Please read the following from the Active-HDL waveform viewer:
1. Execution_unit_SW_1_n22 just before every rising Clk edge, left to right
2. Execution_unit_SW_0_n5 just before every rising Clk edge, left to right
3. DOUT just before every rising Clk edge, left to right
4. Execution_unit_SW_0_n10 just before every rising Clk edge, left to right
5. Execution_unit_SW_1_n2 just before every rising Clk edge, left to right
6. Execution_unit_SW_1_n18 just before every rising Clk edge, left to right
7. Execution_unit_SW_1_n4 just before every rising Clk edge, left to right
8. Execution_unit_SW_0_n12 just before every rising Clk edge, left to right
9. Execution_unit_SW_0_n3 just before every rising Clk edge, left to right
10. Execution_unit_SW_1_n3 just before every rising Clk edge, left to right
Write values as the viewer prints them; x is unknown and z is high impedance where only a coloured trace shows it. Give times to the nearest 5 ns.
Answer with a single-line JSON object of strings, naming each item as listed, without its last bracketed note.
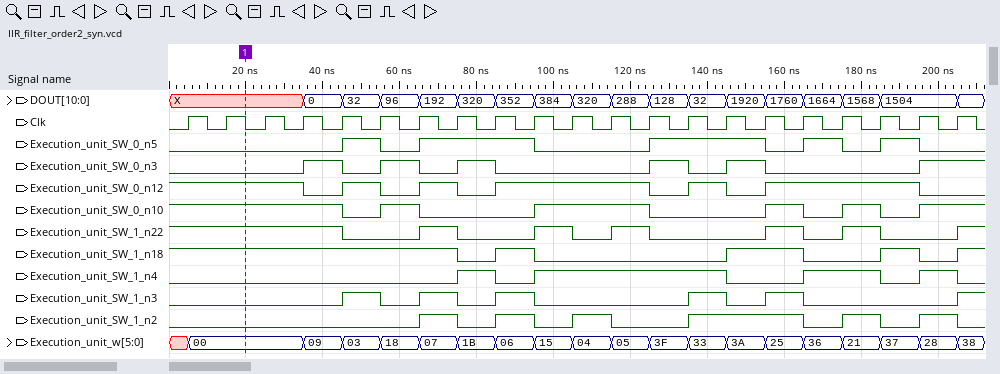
{"Execution_unit_SW_1_n22 just before every rising Clk edge, left to right": "1 1 1 1 1 0 0 1 0 0 1 0 1 0 0 0 1 0 1 0 0", "Execution_unit_SW_0_n5 just before every rising Clk edge, left to right": "0 0 0 0 0 1 0 1 1 1 0 0 0 1 1 1 0 1 0 1 0", "DOUT just before every rising Clk edge, left to right": "X, X, X, X, 0, 32, 96, 192, 320, 352, 384, 320, 288, 128, 32, 1920, 1760, 1664, 1568, 1504, 1504", "Execution_unit_SW_0_n10 just before every rising Clk edge, left to right": "1 1 1 1 1 0 1 0 0 0 1 1 1 0 0 0 1 0 1 0 1", "Execution_unit_SW_1_n2 just before every rising Clk edge, left to right": "0 0 0 0 0 0 0 1 0 1 0 1 0 0 1 1 1 0 1 0 1", "Execution_unit_SW_1_n18 just before every rising Clk edge, left to right": "1 1 1 1 1 1 1 1 0 1 0 0 0 0 0 1 1 0 0 1 0", "Execution_unit_SW_1_n4 just before every rising Clk edge, left to right": "0 0 0 0 0 0 0 0 1 0 1 1 1 1 1 0 0 1 1 0 1", "Execution_unit_SW_0_n12 just before every rising Clk edge, left to right": "1 1 1 1 0 1 0 1 0 1 1 1 1 0 1 0 1 1 1 1 0", "Execution_unit_SW_0_n3 just before every rising Clk edge, left to right": "0 0 0 0 1 0 1 0 1 0 0 0 0 1 0 1 0 0 0 0 1", "Execution_unit_SW_1_n3 just before every rising Clk edge, left to right": "0 0 0 0 0 1 0 1 0 1 0 0 0 0 1 0 1 0 0 0 0"}
